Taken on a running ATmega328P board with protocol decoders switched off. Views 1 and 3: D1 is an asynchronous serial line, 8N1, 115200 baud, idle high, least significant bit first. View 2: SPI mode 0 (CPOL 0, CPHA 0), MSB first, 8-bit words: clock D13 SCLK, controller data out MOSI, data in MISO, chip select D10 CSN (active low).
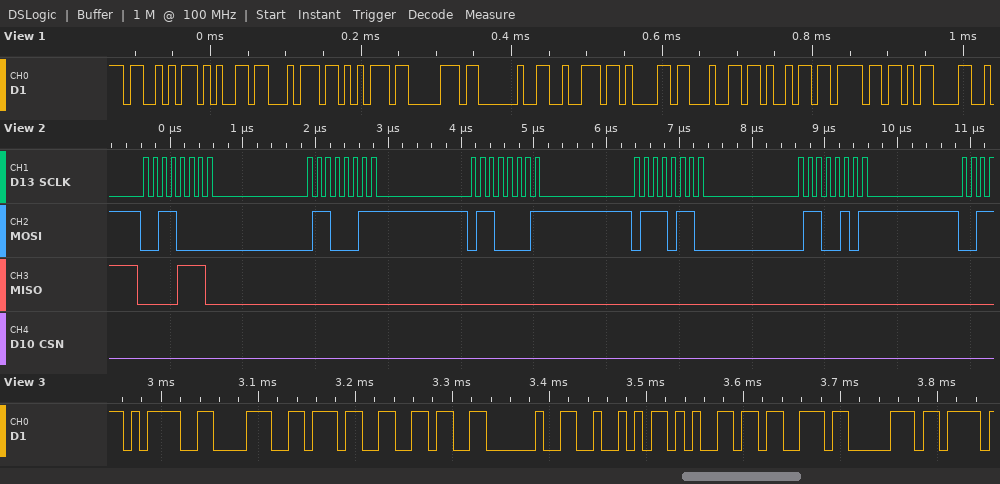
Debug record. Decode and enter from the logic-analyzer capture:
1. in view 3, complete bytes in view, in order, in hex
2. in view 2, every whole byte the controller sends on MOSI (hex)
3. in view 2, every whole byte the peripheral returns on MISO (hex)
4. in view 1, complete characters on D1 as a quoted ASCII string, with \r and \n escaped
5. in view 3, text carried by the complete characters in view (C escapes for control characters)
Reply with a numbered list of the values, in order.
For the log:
1. 3D 38 37 36 20 52 65 73 70
2. 30 63 61 76 65
3. 0E 00 00 00 00
4. "Setup radio\r"
5. "=876 Resp"
